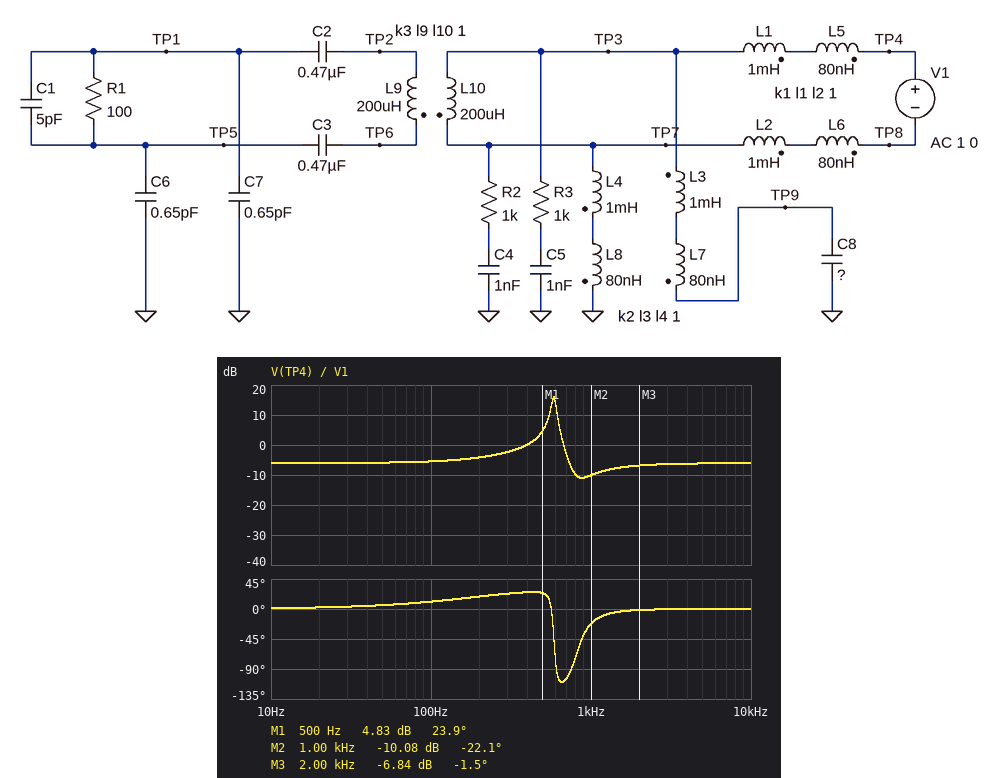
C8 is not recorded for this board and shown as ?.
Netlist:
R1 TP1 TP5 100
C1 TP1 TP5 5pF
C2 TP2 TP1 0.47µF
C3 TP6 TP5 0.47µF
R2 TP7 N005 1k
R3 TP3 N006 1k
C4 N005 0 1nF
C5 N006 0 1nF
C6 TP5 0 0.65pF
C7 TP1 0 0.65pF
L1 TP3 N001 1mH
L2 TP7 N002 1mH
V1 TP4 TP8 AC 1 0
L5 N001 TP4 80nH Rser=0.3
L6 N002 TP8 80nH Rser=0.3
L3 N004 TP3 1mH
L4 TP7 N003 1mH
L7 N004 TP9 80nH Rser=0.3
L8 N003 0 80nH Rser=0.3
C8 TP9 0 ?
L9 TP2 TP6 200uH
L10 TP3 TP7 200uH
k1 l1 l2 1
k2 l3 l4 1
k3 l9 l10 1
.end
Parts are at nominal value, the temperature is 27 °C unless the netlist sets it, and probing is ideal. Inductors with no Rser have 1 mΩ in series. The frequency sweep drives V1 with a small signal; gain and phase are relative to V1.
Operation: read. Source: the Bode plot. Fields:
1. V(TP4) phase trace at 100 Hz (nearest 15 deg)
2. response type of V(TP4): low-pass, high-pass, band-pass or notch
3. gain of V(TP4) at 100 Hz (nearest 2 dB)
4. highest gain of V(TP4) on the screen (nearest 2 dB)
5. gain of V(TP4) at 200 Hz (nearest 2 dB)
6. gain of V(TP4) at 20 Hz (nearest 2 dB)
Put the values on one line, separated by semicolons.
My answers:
15 deg; band-pass; -6 dB; 16 dB; -4 dB; -6 dB
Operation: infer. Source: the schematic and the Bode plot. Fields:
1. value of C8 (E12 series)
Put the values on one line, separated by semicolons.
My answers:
18 µF
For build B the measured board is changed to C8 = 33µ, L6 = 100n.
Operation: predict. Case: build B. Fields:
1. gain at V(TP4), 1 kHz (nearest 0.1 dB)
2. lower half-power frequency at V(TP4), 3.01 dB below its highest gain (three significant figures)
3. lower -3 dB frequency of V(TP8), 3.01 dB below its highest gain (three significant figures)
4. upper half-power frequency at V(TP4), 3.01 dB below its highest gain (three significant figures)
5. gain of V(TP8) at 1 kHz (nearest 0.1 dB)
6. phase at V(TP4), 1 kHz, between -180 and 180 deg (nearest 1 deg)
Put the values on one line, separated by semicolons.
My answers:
-7.7 dB; 412 Hz; 417 Hz; 447 Hz; -4.5 dB; -7 deg
